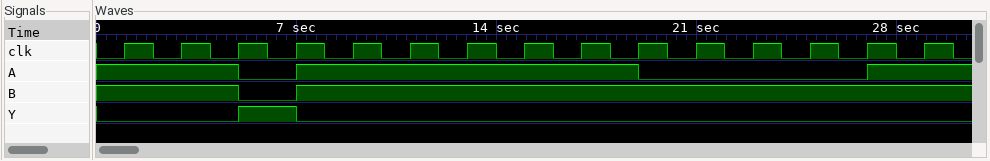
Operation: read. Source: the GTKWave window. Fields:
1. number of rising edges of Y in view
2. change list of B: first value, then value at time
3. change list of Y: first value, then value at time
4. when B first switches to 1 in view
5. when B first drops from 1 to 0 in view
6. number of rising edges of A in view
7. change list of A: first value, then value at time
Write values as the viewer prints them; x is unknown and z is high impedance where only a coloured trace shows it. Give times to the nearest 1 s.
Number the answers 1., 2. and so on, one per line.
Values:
1. 1
2. 1, 0 at 5 s, 1 at 7 s
3. 0, 1 at 5 s, 0 at 7 s
4. 7 s
5. 5 s
6. 2
7. 1, 0 at 5 s, 1 at 7 s, 0 at 19 s, 1 at 27 s
